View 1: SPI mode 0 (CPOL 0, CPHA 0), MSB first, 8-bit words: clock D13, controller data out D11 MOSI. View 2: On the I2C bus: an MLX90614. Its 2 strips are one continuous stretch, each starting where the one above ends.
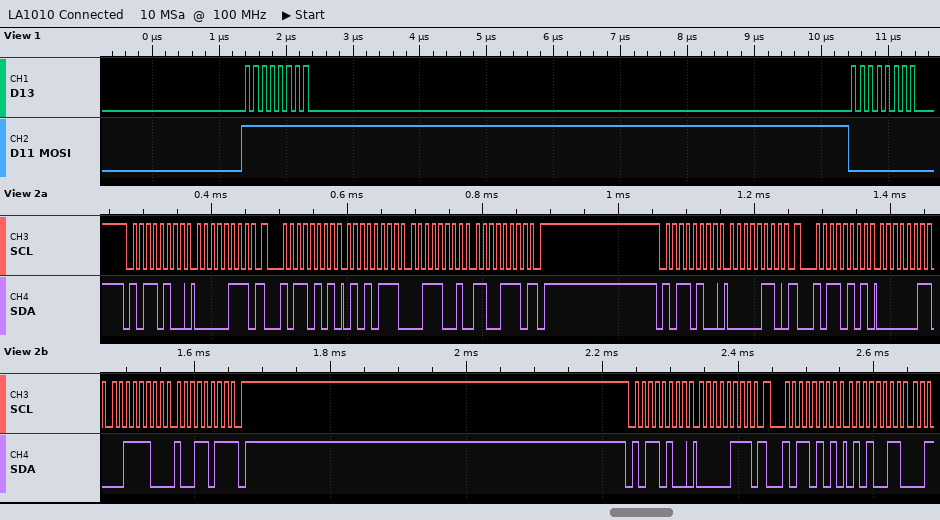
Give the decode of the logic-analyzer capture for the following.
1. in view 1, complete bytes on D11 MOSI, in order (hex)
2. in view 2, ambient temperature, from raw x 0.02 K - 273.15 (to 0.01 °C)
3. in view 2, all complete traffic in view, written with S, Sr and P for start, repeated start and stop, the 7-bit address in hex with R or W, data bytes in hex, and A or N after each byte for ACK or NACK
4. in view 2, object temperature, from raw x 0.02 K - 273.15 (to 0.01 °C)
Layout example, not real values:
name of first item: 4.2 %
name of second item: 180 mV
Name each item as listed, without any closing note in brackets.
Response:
in view 1, complete bytes on D11 MOSI, in order: 0xFF 0x00
in view 2, ambient temperature, from raw x 0.02 K - 273.15: 34.11 °C
in view 2, all complete traffic in view, written with S, Sr and P for start, repeated start and stop, the 7-bit address in hex with R or W, data bytes in hex, and A or N after each byte for ACK or NACK: S 5AW A 07 A Sr 5AR A 57 A 39 A CE N P S 5AW A 06 A Sr 5AR A 03 A 3C A 9B N P S 5AW A 07 A Sr 5AR A 53 A
in view 2, object temperature, from raw x 0.02 K - 273.15: 20.43 °C
